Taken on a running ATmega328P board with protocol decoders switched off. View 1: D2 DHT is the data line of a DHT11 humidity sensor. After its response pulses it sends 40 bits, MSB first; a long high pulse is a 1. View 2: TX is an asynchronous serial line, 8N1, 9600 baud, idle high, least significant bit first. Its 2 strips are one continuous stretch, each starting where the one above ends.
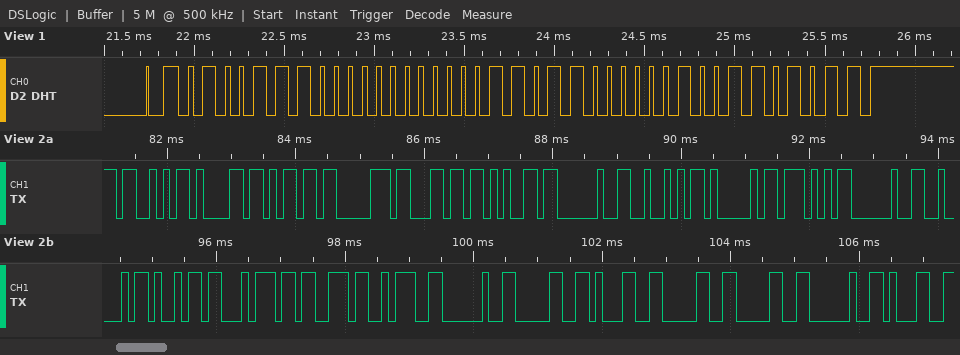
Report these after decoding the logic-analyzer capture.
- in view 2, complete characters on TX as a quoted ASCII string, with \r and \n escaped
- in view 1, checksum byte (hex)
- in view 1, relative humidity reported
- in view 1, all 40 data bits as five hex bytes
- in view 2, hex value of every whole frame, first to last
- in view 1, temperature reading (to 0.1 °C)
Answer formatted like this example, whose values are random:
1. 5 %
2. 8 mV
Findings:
1. "Sample RAW Bits: 0100 1"
2. 0x6B
3. 78 %
4. 4E 00 1B 02 6B
5. 53 61 6D 70 6C 65 20 52 41 57 20 42 69 74 73 3A 20 30 31 30 30 20 31
6. 27.2 °C
